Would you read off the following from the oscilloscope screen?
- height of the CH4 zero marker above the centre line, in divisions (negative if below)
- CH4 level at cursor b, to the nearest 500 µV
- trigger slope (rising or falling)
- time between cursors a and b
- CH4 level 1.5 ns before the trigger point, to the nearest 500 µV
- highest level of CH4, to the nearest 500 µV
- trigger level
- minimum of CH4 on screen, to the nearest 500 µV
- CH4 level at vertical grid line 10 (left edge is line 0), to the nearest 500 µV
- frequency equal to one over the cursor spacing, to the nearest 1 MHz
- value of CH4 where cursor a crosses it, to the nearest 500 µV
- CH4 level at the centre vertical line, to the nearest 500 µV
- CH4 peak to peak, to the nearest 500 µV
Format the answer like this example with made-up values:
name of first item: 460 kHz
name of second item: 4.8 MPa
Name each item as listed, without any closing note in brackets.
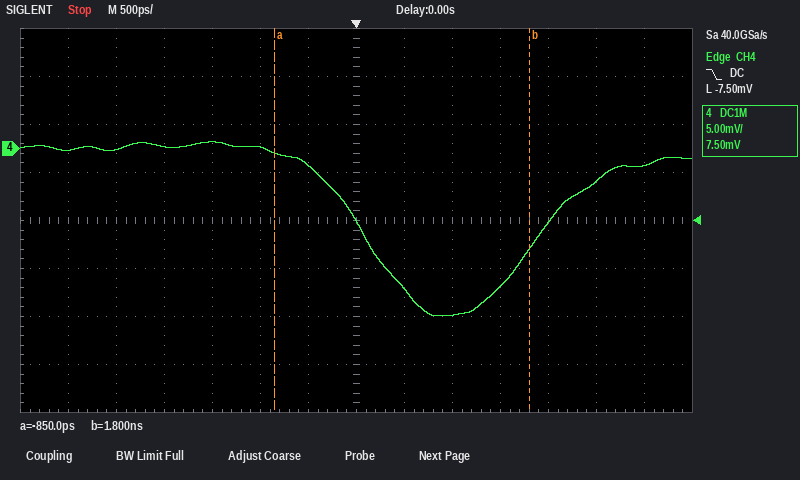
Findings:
height of the CH4 zero marker above the centre line, in divisions: +1.5 div
CH4 level at cursor b, to the nearest 500 µV: -10.5 mV
trigger slope: falling
time between cursors a and b: 2.65 ns
CH4 level 1.5 ns before the trigger point, to the nearest 500 µV: 500 µV
highest level of CH4, to the nearest 500 µV: 500 µV
trigger level: -7.50 mV
minimum of CH4 on screen, to the nearest 500 µV: -17.5 mV
CH4 level at vertical grid line 10 (left edge is line 0), to the nearest 500 µV: -14.5 mV
frequency equal to one over the cursor spacing, to the nearest 1 MHz: 377 MHz
value of CH4 where cursor a crosses it, to the nearest 500 µV: -500 µV
CH4 level at the centre vertical line, to the nearest 500 µV: -7.5 mV
CH4 peak to peak, to the nearest 500 µV: 18.0 mV
